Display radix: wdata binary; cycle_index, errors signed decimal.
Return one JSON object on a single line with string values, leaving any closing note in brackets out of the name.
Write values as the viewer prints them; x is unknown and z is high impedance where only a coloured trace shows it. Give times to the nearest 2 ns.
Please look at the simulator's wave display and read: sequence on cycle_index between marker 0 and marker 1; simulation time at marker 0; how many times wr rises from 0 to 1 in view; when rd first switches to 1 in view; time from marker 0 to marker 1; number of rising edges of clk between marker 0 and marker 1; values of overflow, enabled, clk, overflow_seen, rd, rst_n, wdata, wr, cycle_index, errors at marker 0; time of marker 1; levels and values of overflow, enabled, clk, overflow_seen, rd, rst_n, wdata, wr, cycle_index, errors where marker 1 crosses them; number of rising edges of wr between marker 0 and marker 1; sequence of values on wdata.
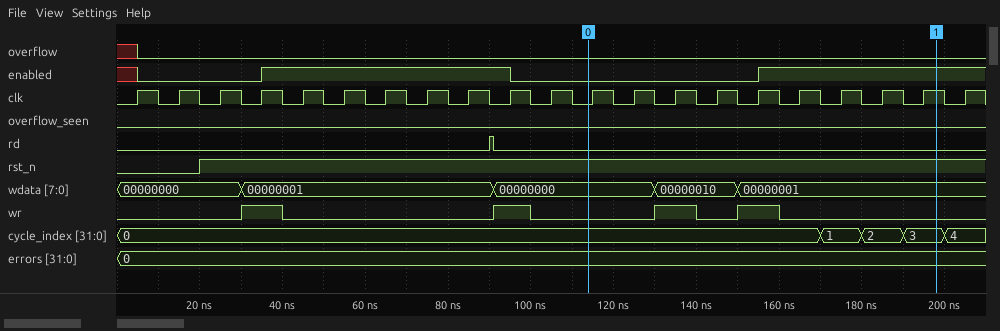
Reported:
{"sequence on cycle_index between marker 0 and marker 1": "0, 1, 2, 3", "simulation time at marker 0": "114 ns", "how many times wr rises from 0 to 1 in view": "4", "when rd first switches to 1 in view": "90 ns", "time from marker 0 to marker 1": "84 ns", "number of rising edges of clk between marker 0 and marker 1": "9", "values of overflow, enabled, clk, overflow_seen, rd, rst_n, wdata, wr, cycle_index, errors at marker 0": "overflow=0, enabled=0, clk=0, overflow_seen=0, rd=0, rst_n=1, wdata=00000000, wr=0, cycle_index=0, errors=0", "time of marker 1": "198 ns", "levels and values of overflow, enabled, clk, overflow_seen, rd, rst_n, wdata, wr, cycle_index, errors where marker 1 crosses them": "overflow=0, enabled=1, clk=1, overflow_seen=0, rd=0, rst_n=1, wdata=00000001, wr=0, cycle_index=3, errors=0", "number of rising edges of wr between marker 0 and marker 1": "2", "sequence of values on wdata": "00000000, 00000001, 00000000, 00000010, 00000001"}
